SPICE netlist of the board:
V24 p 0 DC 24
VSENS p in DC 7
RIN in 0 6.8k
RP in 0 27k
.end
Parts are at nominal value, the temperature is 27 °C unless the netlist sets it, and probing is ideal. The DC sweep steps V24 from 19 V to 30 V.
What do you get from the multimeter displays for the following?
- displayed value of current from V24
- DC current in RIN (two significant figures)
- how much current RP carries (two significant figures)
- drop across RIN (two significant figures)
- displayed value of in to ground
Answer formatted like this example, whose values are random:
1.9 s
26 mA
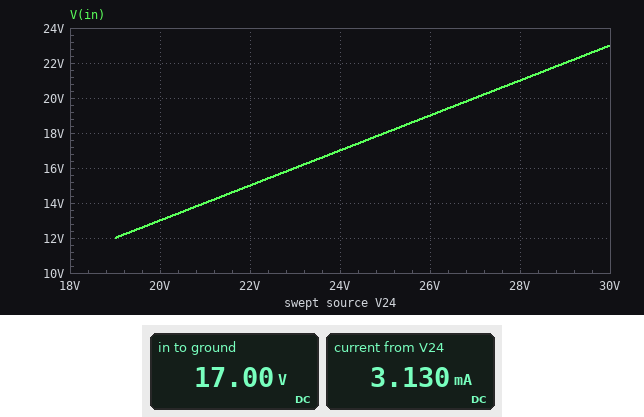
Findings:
3.130 mA
2.5 mA
630 µA
17 V
17.00 V
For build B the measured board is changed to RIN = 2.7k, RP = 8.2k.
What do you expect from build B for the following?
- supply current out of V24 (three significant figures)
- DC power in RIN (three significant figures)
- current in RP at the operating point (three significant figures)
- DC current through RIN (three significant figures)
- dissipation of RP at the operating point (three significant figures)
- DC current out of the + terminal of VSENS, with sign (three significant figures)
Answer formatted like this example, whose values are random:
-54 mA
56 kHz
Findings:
8.37 mA
107 mW
2.07 mA
6.30 mA
35.2 mW
-8.37 mA
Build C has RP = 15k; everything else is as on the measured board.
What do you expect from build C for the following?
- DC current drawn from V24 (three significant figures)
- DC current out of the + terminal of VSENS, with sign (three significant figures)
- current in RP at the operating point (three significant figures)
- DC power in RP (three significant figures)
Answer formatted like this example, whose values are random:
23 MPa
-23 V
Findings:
3.63 mA
-3.63 mA
1.13 mA
19.3 mW
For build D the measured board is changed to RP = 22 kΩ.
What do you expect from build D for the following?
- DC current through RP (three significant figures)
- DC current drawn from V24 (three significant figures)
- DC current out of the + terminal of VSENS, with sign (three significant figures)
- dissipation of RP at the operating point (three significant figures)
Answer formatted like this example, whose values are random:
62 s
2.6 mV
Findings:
773 µA
3.27 mA
-3.27 mA
13.1 mW
